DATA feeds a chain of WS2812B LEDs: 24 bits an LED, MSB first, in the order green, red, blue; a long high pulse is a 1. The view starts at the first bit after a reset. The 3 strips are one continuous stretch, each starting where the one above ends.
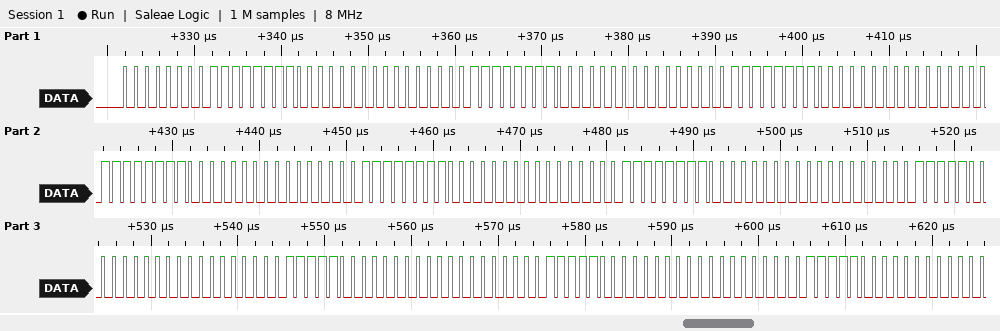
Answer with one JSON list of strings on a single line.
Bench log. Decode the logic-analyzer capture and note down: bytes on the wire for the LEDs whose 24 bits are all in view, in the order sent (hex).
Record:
["00 FF 00 00 FF 00 00 FF 00 00 FF 00 00 FF 00 00 FF 00 00 1F 00 00 1F 00 00 1F 00 00 1F 00"]
